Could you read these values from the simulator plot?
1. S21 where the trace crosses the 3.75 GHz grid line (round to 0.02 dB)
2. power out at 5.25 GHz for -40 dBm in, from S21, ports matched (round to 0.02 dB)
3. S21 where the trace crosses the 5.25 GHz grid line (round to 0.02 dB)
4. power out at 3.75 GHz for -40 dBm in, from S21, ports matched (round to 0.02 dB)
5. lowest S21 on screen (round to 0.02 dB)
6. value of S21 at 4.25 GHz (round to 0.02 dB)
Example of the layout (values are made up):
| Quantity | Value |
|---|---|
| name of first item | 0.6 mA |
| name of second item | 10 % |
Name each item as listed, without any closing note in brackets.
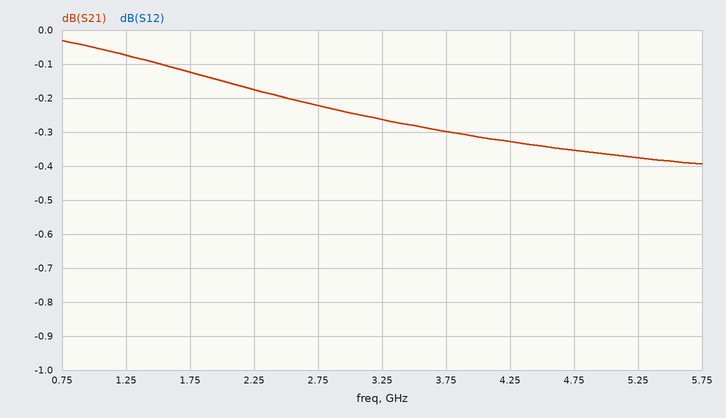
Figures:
| Quantity | Value |
|---|---|
| S21 where the trace crosses the 3.75 GHz grid line | -0.30 dB |
| power out at 5.25 GHz for -40 dBm in, from S21, ports matched | -40.38 dBm |
| S21 where the trace crosses the 5.25 GHz grid line | -0.38 dB |
| power out at 3.75 GHz for -40 dBm in, from S21, ports matched | -40.30 dBm |
| lowest S21 on screen | -0.40 dB |
| value of S21 at 4.25 GHz | -0.32 dB |
